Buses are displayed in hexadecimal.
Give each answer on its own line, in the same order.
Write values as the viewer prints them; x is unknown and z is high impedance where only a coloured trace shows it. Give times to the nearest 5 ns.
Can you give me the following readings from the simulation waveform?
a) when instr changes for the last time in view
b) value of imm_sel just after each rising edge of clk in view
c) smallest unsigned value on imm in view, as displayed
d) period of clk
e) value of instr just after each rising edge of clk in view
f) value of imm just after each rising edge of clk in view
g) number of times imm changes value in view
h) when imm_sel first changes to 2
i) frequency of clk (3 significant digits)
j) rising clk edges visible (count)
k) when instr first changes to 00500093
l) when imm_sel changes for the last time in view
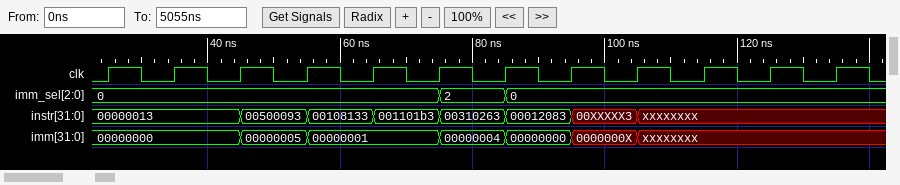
105 ns
0, 0, 0, 0, 0, 2, 0, 0, 0, 0, 0, 0
00000000
10 ns
00000013, 00000013, 00500093, 00108133, 001101b3, 00310263, 00012083, 00XXXXX3, xxxxxxxx, xxxxxxxx, xxxxxxxx, xxxxxxxx
00000000, 00000000, 00000005, 00000001, 00000001, 00000004, 00000000, 0000000X, xxxxxxxx, xxxxxxxx, xxxxxxxx, xxxxxxxx
6
75 ns
100 MHz
12
45 ns
85 ns
